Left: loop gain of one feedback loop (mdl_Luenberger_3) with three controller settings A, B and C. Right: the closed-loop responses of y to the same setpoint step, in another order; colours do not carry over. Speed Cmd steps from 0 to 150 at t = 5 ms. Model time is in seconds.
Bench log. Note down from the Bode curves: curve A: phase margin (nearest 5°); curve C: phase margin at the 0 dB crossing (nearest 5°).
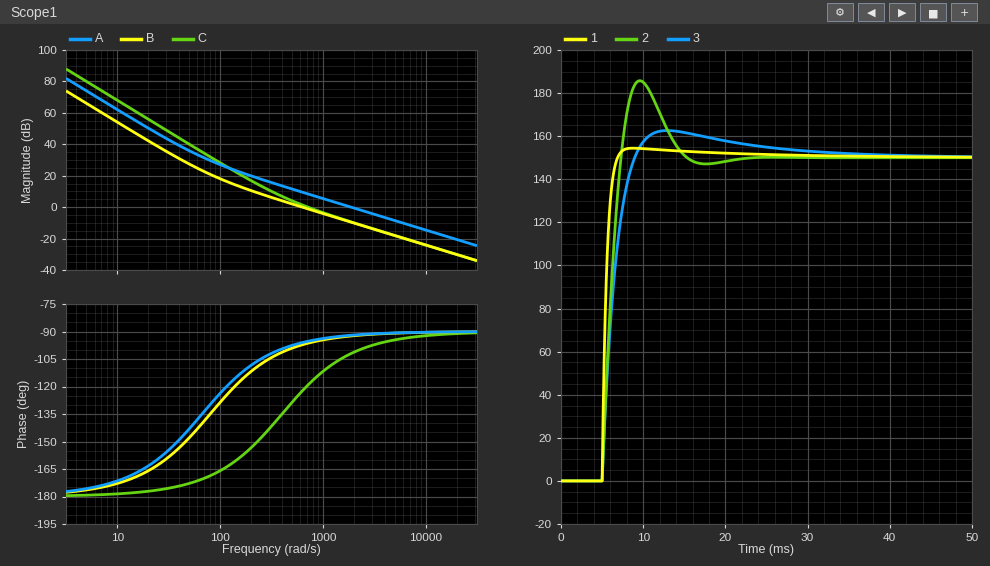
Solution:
90°
60°
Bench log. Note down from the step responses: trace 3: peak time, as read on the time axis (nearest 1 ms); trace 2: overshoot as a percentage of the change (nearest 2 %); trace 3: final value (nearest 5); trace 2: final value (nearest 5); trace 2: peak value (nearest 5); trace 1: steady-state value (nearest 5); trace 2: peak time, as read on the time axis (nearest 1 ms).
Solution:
13 ms
24 %
150
150
185
150
10 ms
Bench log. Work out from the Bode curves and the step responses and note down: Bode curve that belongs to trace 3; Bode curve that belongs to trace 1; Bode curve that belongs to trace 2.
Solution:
B
A
C
